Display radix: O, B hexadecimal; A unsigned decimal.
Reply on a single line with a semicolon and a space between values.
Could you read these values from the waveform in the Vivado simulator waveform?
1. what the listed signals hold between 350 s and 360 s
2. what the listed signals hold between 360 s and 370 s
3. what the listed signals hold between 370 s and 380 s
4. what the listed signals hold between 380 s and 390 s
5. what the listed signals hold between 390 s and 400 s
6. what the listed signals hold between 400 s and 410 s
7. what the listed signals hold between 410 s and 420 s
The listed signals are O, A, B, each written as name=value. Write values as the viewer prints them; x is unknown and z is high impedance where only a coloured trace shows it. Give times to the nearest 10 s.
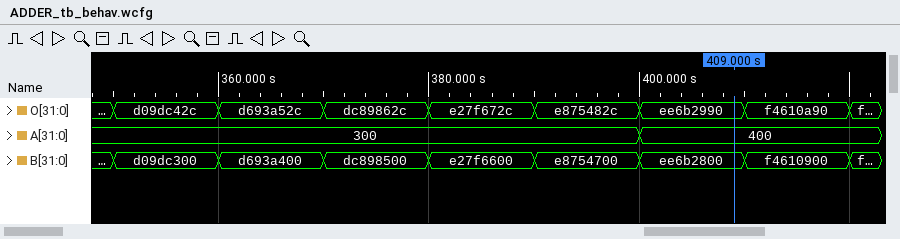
O=d09dc42c, A=300, B=d09dc300; O=d693a52c, A=300, B=d693a400; O=dc89862c, A=300, B=dc898500; O=e27f672c, A=300, B=e27f6600; O=e875482c, A=300, B=e8754700; O=ee6b2990, A=400, B=ee6b2800; O=f4610a90, A=400, B=f4610900
